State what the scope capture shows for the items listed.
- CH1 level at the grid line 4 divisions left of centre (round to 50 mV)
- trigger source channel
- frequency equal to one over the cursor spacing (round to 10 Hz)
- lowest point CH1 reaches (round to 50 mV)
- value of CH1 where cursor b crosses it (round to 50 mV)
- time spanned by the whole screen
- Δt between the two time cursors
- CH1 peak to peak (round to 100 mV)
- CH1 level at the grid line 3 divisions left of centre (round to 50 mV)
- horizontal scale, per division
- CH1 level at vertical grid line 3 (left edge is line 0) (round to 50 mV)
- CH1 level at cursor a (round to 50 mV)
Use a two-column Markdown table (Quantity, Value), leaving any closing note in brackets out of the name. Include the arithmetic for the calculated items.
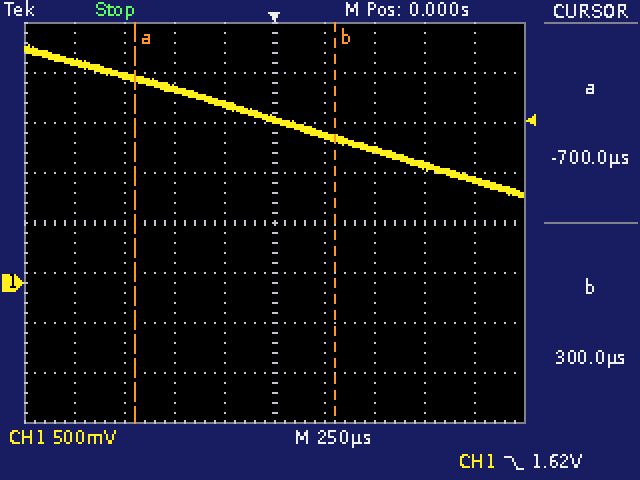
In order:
| Quantity | Value |
|---|---|
| CH1 level at the grid line 4 divisions left of centre | 2.20 V |
| trigger source channel | CH1 |
| frequency equal to one over the cursor spacing | 1 / 1.000 ms ≈ 1.00 kHz |
| lowest point CH1 reaches | 850 mV |
| value of CH1 where cursor b crosses it | 1.45 V |
| time spanned by the whole screen | 2.5 ms |
| Δt between the two time cursors | 300 µs − (-700 µs) = 1.000 ms |
| CH1 peak to peak | 1.50 V |
| CH1 level at the grid line 3 divisions left of centre | 2.05 V |
| horizontal scale, per division | 250 µs |
| CH1 level at vertical grid line 3 (left edge is line 0) | 1.95 V |
| CH1 level at cursor a | 2.05 V |
